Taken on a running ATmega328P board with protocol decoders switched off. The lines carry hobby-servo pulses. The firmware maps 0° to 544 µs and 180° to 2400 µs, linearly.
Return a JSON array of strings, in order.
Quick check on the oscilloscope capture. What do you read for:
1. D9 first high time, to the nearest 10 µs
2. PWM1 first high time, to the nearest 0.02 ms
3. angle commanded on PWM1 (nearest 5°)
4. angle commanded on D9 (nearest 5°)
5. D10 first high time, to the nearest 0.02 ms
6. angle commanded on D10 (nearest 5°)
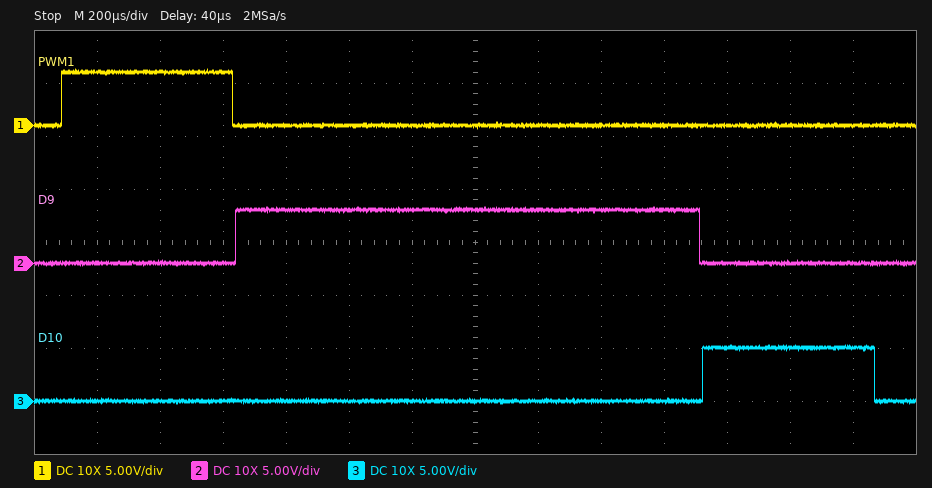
["1470 µs", "0.54 ms", "0°", "90°", "0.54 ms", "0°"]
